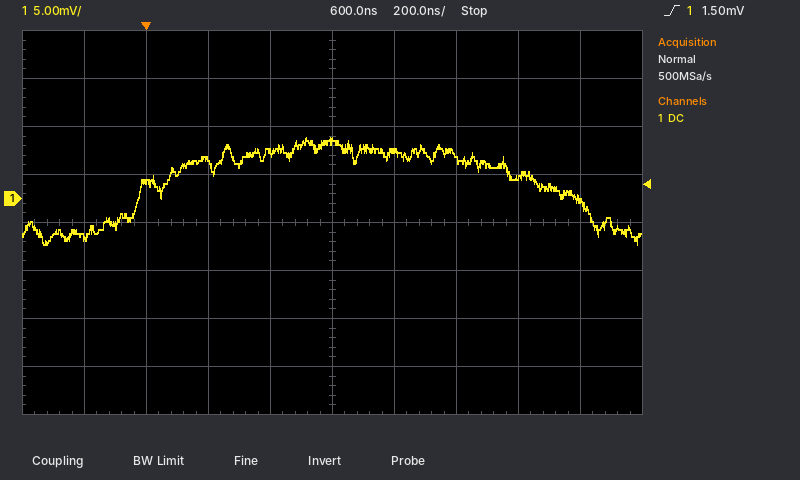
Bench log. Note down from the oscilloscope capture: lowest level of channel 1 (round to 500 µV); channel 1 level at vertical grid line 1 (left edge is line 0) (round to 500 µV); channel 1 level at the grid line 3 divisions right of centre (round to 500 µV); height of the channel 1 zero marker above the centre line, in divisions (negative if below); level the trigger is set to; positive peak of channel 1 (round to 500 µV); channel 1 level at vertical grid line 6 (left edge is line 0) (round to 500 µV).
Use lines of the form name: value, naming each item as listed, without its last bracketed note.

lowest level of channel 1: -5.0 mV
channel 1 level at vertical grid line 1 (left edge is line 0): -4.0 mV
channel 1 level at the grid line 3 divisions right of centre: 2.0 mV
height of the channel 1 zero marker above the centre line, in divisions: +0.5 div
level the trigger is set to: 1.50 mV
positive peak of channel 1: 6.5 mV
channel 1 level at vertical grid line 6 (left edge is line 0): 5.0 mV
